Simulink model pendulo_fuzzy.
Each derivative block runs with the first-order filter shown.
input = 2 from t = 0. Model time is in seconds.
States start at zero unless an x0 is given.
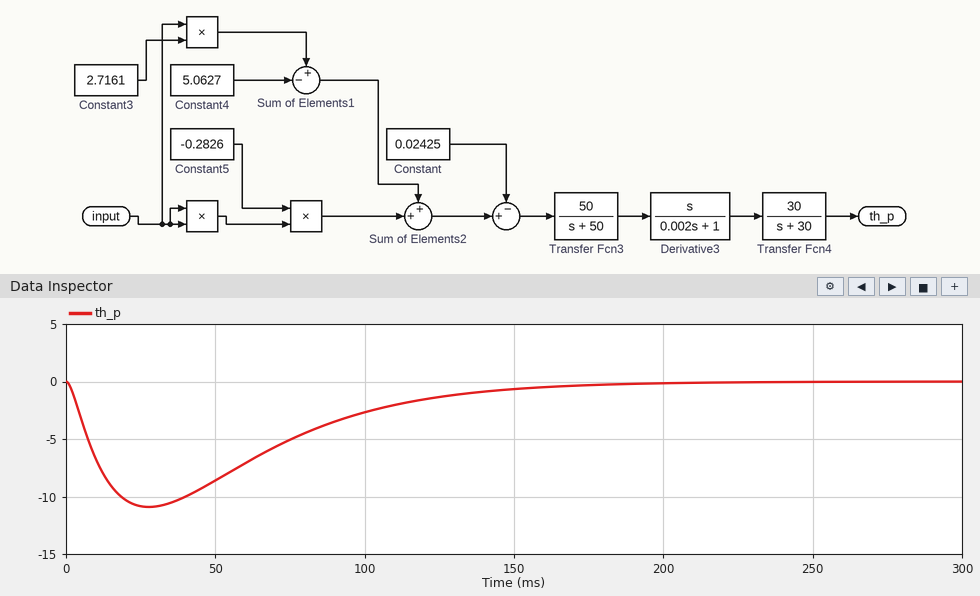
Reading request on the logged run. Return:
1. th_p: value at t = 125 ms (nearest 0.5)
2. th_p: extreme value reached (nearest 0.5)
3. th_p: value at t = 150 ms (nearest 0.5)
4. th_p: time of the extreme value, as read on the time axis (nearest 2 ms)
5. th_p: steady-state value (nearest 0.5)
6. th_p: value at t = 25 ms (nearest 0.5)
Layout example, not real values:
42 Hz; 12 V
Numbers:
-1.5; -11.0; -0.5; 28 ms; 0.0; -11.0
